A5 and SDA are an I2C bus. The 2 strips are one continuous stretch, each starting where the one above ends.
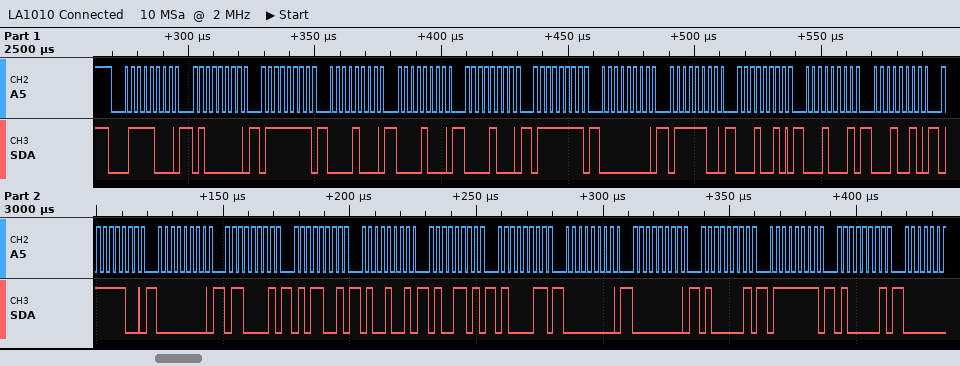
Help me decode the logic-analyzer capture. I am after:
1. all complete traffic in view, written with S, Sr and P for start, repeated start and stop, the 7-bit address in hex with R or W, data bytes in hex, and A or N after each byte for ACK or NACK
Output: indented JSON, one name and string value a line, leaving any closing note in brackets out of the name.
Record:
{
  "all complete traffic in view, written with S, Sr and P for start, repeated start and stop, the 7-bit address in hex with R or W, data bytes in hex, and A or N after each byte for ACK or NACK": "S 3CW A 40 A 7F A 08 A 08 A 08 A 7F A 00 A 7C A 12 A 11 A 12 A 7C A 00 A 61 A 59 A 49 A 4D A 43 A 00 A 00 A 41 A 7F A 41 A"
}
